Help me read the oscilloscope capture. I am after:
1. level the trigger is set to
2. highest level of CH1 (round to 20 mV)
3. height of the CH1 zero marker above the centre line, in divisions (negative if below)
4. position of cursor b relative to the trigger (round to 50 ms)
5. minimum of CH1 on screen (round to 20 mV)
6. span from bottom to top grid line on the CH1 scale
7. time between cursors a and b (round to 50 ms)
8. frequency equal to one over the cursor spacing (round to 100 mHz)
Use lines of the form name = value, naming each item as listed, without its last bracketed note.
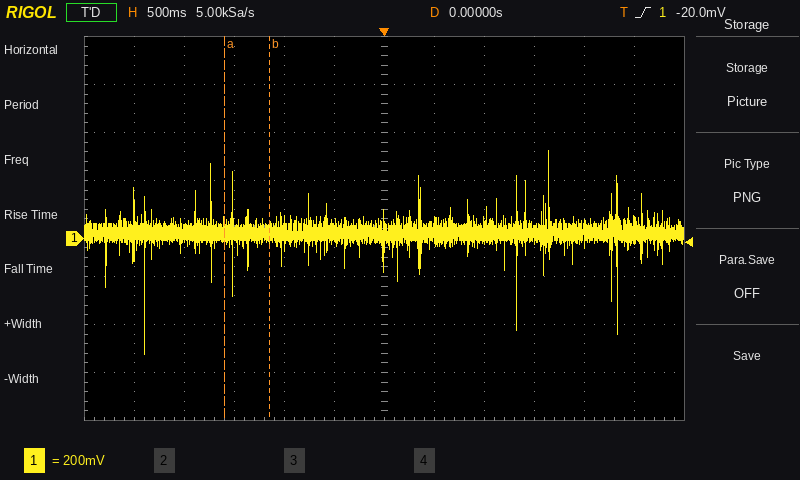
level the trigger is set to = -20.0 mV
highest level of CH1 = 360 mV
height of the CH1 zero marker above the centre line, in divisions = -0.2 div
position of cursor b relative to the trigger = -1.15 s
minimum of CH1 on screen = -480 mV
span from bottom to top grid line on the CH1 scale = 1.6 V
time between cursors a and b = 450 ms
frequency equal to one over the cursor spacing = 2.2 Hz
